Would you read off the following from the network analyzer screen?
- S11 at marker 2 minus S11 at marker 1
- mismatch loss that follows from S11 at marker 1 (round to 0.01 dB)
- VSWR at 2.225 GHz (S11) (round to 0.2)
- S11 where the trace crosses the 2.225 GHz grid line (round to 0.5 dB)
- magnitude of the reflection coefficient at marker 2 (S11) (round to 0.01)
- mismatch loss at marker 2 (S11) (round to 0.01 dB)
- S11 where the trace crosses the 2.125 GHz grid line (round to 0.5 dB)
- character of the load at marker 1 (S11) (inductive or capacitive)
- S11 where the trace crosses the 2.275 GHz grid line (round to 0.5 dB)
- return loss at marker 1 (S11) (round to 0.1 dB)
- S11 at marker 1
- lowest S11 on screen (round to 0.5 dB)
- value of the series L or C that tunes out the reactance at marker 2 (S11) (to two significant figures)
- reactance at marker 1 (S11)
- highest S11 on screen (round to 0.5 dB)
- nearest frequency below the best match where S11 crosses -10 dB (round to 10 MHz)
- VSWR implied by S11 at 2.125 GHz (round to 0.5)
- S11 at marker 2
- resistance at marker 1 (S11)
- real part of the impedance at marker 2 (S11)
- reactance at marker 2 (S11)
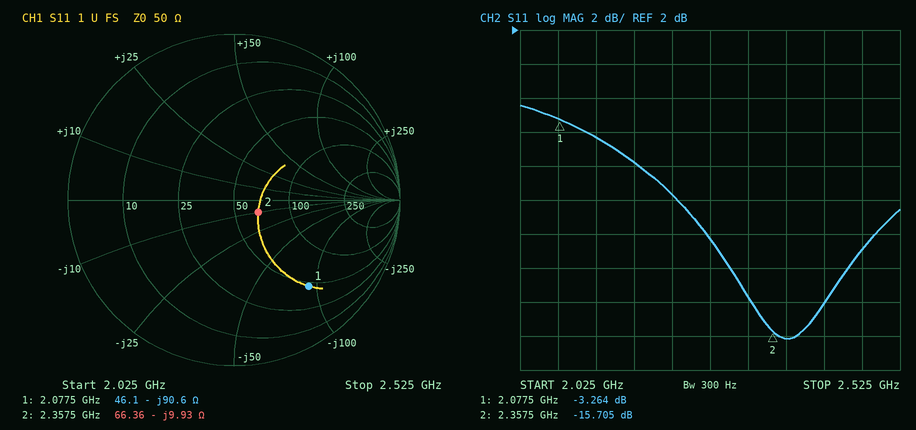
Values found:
-12.441 dB
2.77 dB
2.4
-7.5 dB
0.16
0.12 dB
-4.5 dB
capacitive
-10.5 dB
3.3 dB
-3.264 dB
-16.0 dB
670 pH
-90.6 Ω
-2.5 dB
2.27 GHz
4.0
-15.705 dB
46.1 Ω
66.36 Ω
-9.93 Ω
